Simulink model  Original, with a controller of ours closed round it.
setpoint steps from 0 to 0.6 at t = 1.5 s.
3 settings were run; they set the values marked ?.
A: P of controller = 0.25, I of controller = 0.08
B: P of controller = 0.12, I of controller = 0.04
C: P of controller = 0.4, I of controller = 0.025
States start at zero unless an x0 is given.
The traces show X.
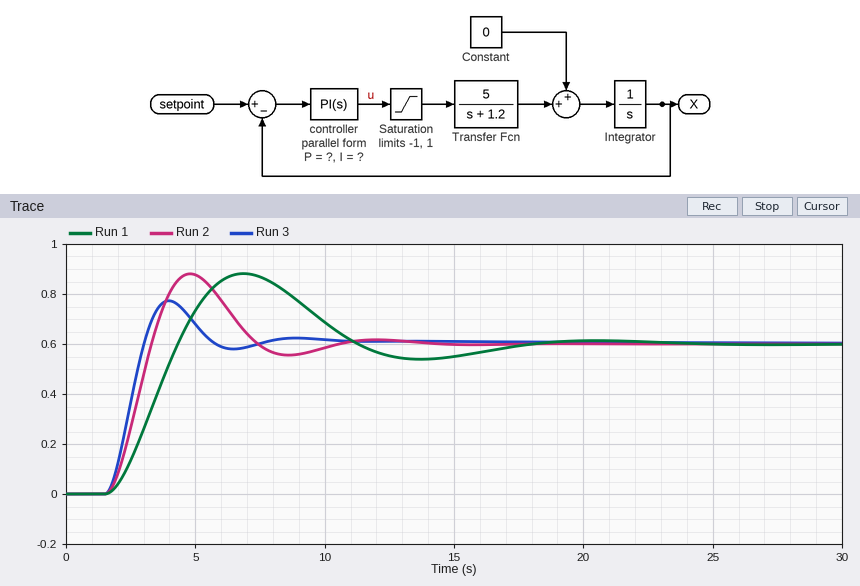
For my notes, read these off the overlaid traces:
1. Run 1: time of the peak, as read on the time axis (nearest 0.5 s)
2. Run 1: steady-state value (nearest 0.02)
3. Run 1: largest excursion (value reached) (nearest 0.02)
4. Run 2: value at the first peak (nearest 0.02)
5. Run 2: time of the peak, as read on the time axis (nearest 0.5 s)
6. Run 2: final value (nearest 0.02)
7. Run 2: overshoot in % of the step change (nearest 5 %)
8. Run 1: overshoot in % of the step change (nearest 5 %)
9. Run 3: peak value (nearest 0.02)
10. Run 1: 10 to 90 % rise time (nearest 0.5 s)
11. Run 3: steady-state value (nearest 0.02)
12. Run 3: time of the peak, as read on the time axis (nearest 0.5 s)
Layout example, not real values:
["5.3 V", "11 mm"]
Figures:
["7.0 s", "0.60", "0.88", "0.88", "5.0 s", "0.60", "45 %", "45 %", "0.78", "2.0 s", "0.60", "4.0 s"]
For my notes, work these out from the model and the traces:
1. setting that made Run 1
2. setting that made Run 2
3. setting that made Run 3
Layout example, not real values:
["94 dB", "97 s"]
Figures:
["B", "A", "C"]
